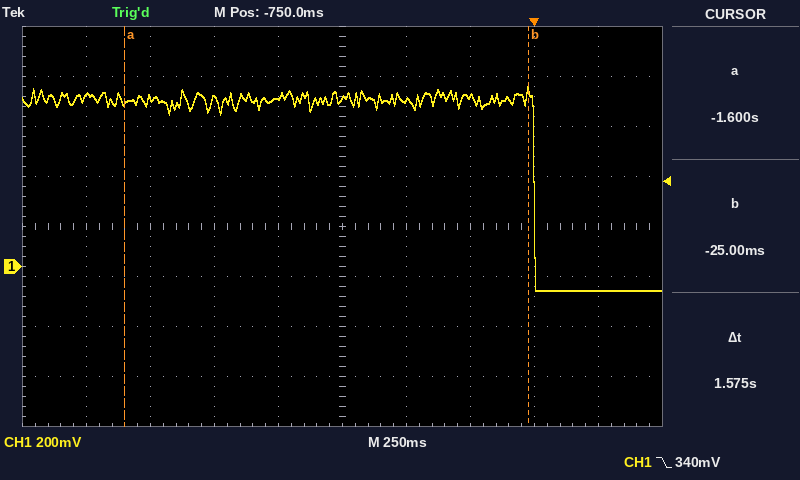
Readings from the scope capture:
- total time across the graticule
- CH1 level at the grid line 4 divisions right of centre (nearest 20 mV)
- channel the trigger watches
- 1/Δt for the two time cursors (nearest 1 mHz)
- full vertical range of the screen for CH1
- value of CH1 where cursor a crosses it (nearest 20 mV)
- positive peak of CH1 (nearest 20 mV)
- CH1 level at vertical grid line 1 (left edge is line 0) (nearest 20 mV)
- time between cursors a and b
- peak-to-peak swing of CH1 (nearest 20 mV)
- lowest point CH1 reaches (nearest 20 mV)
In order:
2.5 s
-100 mV
CH1
635 mHz
1.6 V
660 mV
720 mV
680 mV
1.575 s
820 mV
-100 mV
